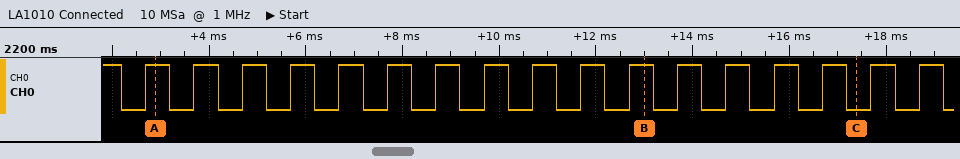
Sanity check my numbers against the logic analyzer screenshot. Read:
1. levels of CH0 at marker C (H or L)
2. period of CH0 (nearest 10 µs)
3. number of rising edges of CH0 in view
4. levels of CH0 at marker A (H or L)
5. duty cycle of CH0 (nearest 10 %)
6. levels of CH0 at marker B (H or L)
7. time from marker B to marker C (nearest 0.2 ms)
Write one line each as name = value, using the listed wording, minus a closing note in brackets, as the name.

levels of CH0 at marker C = CH0=L
period of CH0 = 1000 µs
number of rising edges of CH0 in view = 17
levels of CH0 at marker A = CH0=H
duty cycle of CH0 = 50 %
levels of CH0 at marker B = CH0=H
time from marker B to marker C = 4.4 ms
